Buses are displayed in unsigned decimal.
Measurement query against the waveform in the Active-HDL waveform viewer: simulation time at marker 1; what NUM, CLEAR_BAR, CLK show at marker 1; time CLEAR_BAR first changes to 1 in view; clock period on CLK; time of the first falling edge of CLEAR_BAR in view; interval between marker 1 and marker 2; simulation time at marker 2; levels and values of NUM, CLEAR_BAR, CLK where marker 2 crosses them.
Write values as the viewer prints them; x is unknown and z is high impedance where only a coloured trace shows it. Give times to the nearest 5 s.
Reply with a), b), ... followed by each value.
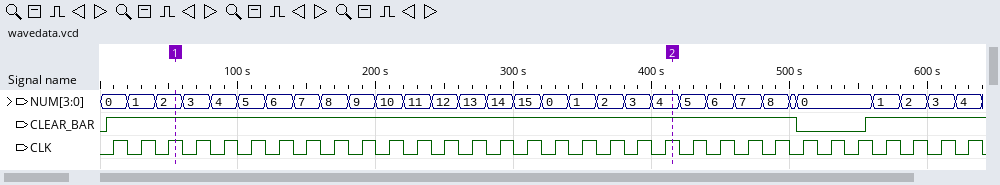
a) 55 s
b) NUM=2, CLEAR_BAR=1, CLK=1
c) 5 s
d) 20 s
e) 505 s
f) 360 s
g) 415 s
h) NUM=4, CLEAR_BAR=1, CLK=1
